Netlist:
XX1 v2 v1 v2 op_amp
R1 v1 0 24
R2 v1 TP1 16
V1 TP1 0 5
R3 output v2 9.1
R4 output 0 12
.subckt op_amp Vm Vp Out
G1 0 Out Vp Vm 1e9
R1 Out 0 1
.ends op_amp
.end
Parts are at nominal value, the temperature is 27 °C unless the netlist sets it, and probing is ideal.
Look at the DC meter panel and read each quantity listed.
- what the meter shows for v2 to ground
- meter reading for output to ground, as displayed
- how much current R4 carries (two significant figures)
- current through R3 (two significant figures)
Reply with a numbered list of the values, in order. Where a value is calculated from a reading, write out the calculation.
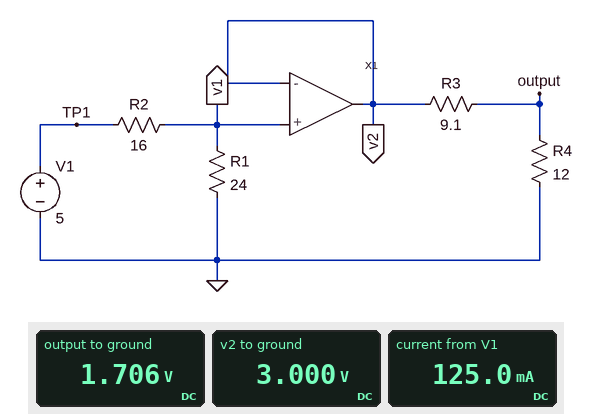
1. 3.000 V
2. 1.706 V
3. (1.706 V) / 12 Ω = 140 mA
4. (3 V - 1.706 V) / 9.1 Ω = 140 mA
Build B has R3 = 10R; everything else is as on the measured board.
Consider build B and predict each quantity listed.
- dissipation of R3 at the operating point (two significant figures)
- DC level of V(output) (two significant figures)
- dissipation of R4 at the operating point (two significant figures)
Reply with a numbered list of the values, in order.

1. 190 mW
2. 1.6 V
3. 220 mW
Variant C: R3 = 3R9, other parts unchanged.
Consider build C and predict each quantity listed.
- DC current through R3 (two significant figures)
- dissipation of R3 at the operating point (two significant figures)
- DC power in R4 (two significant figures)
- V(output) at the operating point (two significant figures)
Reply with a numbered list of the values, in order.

1. 190 mA
2. 140 mW
3. 430 mW
4. 2.3 V
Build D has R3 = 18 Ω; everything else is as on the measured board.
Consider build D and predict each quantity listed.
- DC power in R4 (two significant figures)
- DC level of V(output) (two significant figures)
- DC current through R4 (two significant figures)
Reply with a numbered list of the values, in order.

1. 120 mW
2. 1.2 V
3. 100 mA
